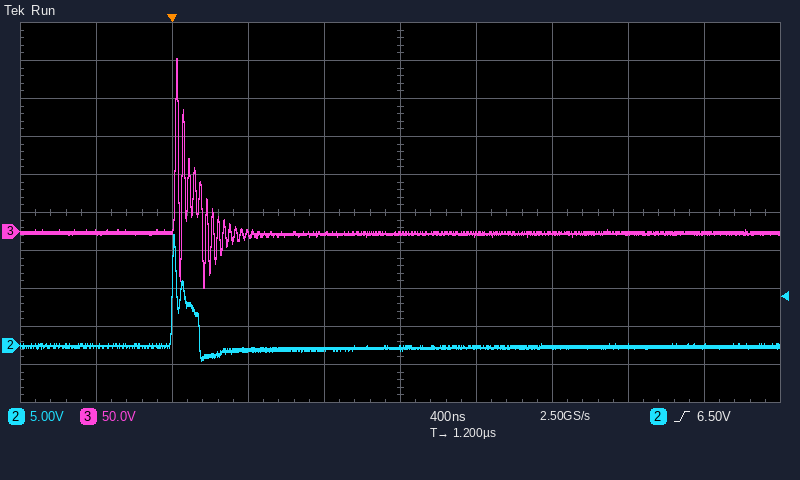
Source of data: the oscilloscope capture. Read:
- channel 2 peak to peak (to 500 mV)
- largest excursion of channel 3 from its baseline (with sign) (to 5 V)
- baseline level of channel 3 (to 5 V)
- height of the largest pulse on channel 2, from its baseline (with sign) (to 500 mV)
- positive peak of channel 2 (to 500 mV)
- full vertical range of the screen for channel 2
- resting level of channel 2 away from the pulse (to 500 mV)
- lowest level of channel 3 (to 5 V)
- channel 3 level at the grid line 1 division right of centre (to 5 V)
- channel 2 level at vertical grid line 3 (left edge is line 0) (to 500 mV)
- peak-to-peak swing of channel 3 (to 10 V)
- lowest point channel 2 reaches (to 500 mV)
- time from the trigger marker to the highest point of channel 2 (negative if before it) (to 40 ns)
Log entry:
16.5 V
+230 V
0 V
+14.5 V
14.5 V
50 V
0.0 V
-75 V
-5 V
-500 mV
300 V
-2.0 V
0 ns
